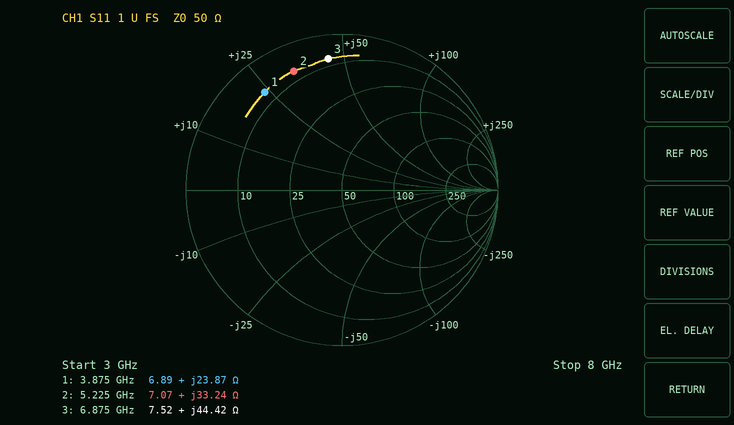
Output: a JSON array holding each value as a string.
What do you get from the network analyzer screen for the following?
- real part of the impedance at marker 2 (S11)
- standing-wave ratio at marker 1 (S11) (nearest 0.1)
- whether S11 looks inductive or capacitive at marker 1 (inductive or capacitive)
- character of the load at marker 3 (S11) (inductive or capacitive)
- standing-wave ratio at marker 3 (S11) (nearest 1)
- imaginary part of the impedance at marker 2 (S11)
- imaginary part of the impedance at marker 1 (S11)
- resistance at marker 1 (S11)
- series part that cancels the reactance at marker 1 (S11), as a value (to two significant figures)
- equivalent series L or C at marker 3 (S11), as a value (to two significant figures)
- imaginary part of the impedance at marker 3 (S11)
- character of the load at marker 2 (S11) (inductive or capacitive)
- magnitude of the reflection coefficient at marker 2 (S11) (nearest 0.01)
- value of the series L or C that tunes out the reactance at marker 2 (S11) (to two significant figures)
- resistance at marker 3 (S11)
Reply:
["7.07 Ω", "8.9", "inductive", "inductive", "12", "+33.24 Ω", "+23.87 Ω", "6.89 Ω", "1.7 pF", "1.0 nH", "+44.42 Ω", "inductive", "0.82", "920 fF", "7.52 Ω"]
